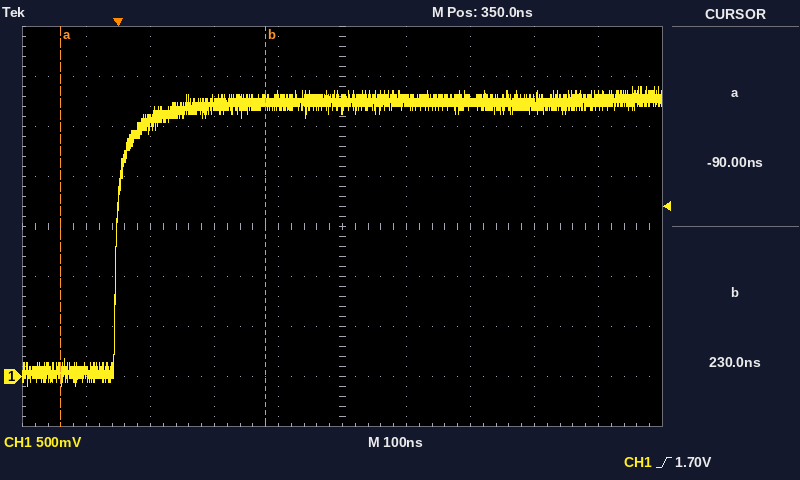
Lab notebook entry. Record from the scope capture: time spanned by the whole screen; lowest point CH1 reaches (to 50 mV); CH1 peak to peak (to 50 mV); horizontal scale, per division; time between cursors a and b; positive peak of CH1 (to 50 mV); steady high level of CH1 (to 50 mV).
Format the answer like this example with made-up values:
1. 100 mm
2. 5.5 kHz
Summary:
1. 1 µs
2. -100 mV
3. 3.00 V
4. 100 ns
5. 320 ns
6. 2.90 V
7. 2.75 V
